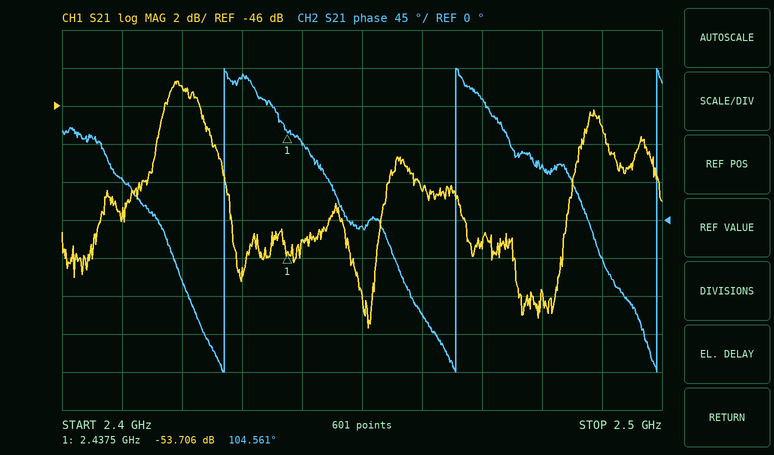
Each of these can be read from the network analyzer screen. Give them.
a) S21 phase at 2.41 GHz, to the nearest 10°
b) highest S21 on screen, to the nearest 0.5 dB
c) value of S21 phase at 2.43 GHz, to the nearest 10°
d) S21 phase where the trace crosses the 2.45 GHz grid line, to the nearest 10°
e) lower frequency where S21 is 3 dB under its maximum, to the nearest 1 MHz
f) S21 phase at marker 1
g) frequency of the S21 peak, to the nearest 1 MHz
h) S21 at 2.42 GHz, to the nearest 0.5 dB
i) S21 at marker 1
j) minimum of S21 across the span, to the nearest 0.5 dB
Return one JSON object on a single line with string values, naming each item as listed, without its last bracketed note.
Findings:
{"S21 phase at 2.41 GHz, to the nearest 10°": "50°", "highest S21 on screen, to the nearest 0.5 dB": "-44.5 dB", "value of S21 phase at 2.43 GHz, to the nearest 10°": "170°", "S21 phase where the trace crosses the 2.45 GHz grid line, to the nearest 10°": "-10°", "lower frequency where S21 is 3 dB under its maximum, to the nearest 1 MHz": "2.416 GHz", "S21 phase at marker 1": "104.561°", "frequency of the S21 peak, to the nearest 1 MHz": "2.419 GHz", "S21 at 2.42 GHz, to the nearest 0.5 dB": "-45.0 dB", "S21 at marker 1": "-53.706 dB", "minimum of S21 across the span, to the nearest 0.5 dB": "-57.5 dB"}
